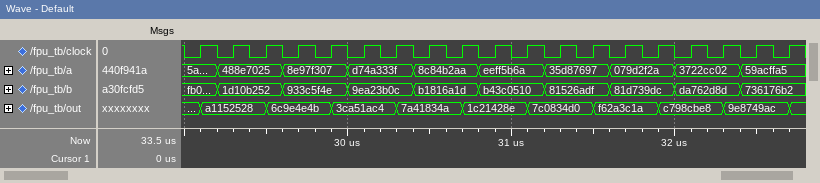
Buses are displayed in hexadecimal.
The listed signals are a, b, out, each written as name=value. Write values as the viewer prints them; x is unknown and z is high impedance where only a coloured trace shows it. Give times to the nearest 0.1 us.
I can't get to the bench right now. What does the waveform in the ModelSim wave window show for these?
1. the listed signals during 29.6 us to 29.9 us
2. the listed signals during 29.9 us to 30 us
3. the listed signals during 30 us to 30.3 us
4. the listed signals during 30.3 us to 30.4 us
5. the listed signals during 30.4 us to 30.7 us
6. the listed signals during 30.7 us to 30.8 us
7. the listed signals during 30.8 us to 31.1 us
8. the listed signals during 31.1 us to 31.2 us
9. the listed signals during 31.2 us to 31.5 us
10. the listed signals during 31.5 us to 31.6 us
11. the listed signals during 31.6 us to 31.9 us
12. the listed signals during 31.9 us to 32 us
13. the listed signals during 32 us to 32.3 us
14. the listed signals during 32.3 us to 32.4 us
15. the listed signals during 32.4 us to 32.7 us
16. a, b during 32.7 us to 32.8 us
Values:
a=8e97f307, b=933c5f4e, out=6c9e4e4b
a=8e97f307, b=933c5f4e, out=3ca51ac4
a=d74a333f, b=9ea23b0c, out=3ca51ac4
a=d74a333f, b=9ea23b0c, out=7a41834a
a=8c84b2aa, b=b1816a1d, out=7a41834a
a=8c84b2aa, b=b1816a1d, out=1c21428e
a=eeff5b6a, b=b43c0510, out=1c21428e
a=eeff5b6a, b=b43c0510, out=7c0834d0
a=35d87697, b=81526adf, out=7c0834d0
a=35d87697, b=81526adf, out=f62a3c1a
a=079d2f2a, b=81d739dc, out=f62a3c1a
a=079d2f2a, b=81d739dc, out=c798cbe8
a=3722cc02, b=da762d8d, out=c798cbe8
a=3722cc02, b=da762d8d, out=9e8749ac
a=59acffa5, b=736176b2, out=9e8749ac
a=59acffa5, b=736176b2
